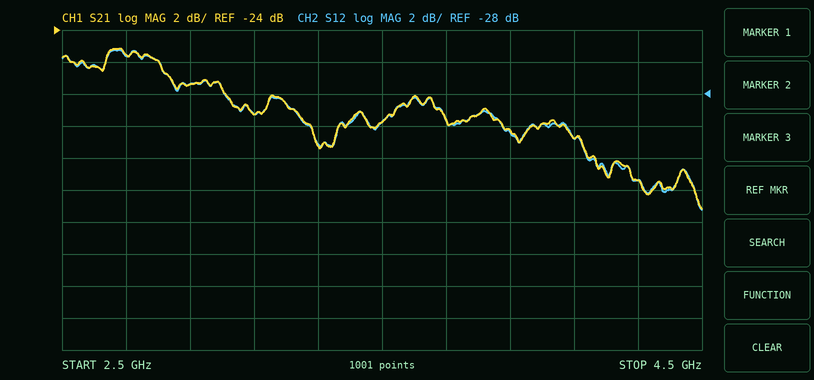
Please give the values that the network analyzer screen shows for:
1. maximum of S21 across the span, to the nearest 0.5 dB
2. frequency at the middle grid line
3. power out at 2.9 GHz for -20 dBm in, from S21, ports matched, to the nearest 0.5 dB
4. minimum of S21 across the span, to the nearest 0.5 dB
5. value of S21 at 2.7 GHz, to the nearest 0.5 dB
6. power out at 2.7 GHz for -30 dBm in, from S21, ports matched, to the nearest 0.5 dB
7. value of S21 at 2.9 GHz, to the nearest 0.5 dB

-25.0 dB
3.5 GHz
-47.5 dBm
-35.0 dB
-25.5 dB
-55.5 dBm
-27.5 dB
